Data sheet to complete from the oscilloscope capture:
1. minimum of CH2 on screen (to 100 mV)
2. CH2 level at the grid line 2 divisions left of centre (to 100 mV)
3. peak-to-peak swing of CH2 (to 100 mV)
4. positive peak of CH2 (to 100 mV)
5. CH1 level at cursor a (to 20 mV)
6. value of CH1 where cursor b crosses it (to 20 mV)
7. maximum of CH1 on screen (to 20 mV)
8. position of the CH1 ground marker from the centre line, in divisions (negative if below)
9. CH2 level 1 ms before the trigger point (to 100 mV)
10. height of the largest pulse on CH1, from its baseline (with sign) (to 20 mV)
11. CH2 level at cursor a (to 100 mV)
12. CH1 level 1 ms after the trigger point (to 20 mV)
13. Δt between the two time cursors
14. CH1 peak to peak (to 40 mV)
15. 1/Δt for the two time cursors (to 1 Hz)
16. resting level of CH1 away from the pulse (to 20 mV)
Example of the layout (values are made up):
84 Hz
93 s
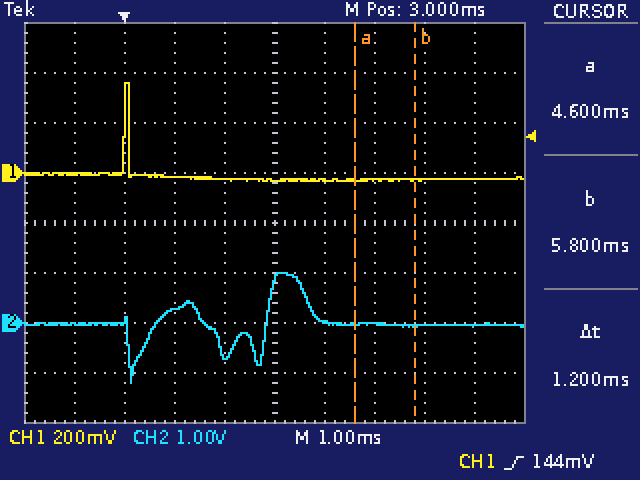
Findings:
-1.2 V
300 mV
2.2 V
1.0 V
-20 mV
-20 mV
360 mV
+1.0 div
0.0 V
+380 mV
0.0 V
-20 mV
1.2 ms
400 mV
833 Hz
-20 mV
